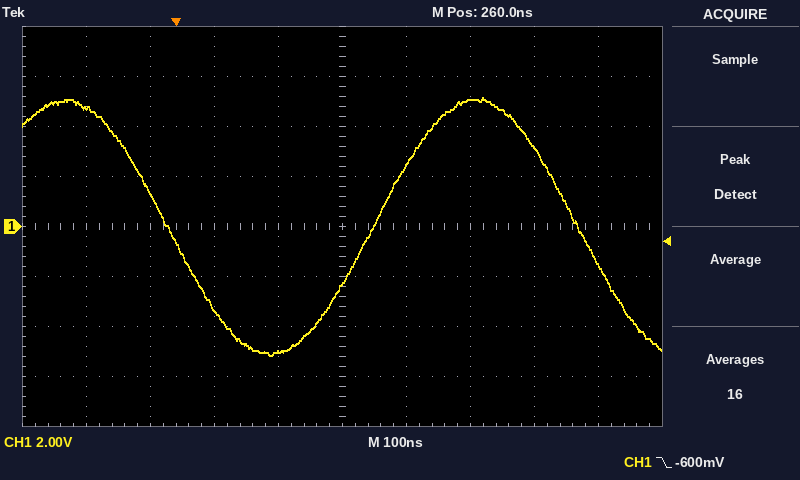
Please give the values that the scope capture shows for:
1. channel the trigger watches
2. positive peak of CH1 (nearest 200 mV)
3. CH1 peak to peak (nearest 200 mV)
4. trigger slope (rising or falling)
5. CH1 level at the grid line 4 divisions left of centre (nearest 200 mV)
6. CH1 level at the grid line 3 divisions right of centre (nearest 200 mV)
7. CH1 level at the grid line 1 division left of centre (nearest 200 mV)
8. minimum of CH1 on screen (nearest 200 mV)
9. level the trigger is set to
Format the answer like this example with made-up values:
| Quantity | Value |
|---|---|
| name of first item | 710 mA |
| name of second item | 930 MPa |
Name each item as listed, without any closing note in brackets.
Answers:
| Quantity | Value |
|---|---|
| channel the trigger watches | CH1 |
| positive peak of CH1 | 5.2 V |
| CH1 peak to peak | 10.4 V |
| trigger slope | falling |
| CH1 level at the grid line 4 divisions left of centre | 4.8 V |
| CH1 level at the grid line 3 divisions right of centre | 3.2 V |
| CH1 level at the grid line 1 division left of centre | -5.0 V |
| minimum of CH1 on screen | -5.2 V |
| level the trigger is set to | -600 mV |
